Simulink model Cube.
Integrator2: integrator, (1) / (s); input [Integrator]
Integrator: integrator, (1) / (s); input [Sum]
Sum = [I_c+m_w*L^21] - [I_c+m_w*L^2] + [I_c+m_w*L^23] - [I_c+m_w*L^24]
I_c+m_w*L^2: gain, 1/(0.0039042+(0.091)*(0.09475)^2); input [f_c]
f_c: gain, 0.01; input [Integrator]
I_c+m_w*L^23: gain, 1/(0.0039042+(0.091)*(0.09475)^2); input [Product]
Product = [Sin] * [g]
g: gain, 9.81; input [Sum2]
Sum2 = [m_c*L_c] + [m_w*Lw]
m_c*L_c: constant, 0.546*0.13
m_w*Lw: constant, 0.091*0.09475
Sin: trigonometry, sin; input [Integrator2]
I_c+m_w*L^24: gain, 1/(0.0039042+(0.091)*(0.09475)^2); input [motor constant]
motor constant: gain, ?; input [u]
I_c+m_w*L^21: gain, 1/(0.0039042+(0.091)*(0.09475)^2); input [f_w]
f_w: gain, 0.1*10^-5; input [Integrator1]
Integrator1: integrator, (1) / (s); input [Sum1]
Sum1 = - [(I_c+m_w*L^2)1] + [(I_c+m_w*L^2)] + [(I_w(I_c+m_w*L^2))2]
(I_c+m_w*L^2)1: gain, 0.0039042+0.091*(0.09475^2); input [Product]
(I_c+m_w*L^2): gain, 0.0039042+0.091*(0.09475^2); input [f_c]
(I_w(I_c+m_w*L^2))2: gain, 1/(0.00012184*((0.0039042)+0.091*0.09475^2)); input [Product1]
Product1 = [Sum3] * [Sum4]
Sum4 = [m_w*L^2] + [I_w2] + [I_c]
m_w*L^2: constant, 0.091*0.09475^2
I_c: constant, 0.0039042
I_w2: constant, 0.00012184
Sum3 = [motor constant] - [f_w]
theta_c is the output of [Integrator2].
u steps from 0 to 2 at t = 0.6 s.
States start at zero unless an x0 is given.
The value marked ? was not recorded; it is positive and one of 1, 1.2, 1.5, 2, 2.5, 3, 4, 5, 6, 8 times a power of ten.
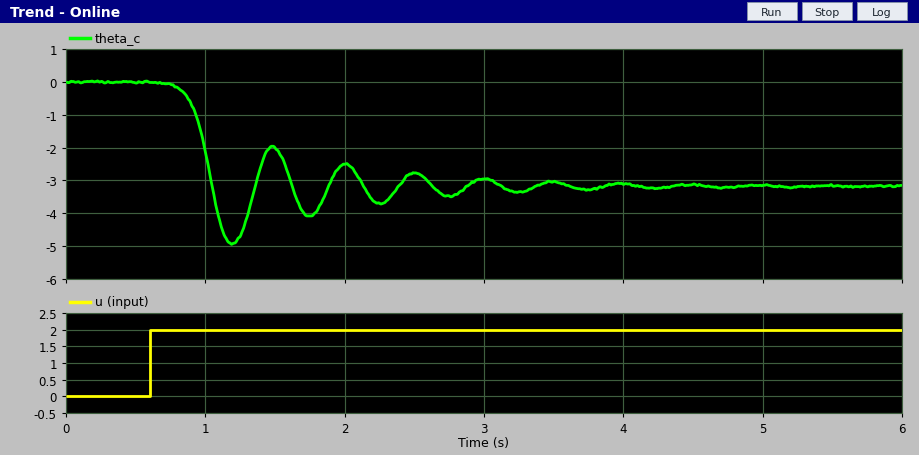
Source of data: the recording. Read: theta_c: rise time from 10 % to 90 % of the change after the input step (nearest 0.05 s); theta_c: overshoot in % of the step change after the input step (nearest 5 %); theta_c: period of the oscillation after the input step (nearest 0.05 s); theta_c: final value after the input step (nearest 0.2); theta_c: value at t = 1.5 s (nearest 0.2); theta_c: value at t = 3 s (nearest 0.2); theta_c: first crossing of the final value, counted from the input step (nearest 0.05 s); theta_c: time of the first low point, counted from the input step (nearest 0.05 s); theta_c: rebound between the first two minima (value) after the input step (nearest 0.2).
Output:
0.20 s
55 %
0.55 s
-3.2
-2.0
-3.0
0.45 s
0.60 s
-2.0
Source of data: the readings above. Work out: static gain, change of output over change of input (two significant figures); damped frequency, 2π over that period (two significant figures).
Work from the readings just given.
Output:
-1.6
11 rad/s
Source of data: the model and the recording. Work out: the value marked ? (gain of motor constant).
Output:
0.015
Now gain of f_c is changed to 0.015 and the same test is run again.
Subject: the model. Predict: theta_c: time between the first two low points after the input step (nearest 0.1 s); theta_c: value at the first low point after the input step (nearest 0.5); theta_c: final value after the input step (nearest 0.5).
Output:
0.5 s
-4.5
-3.0
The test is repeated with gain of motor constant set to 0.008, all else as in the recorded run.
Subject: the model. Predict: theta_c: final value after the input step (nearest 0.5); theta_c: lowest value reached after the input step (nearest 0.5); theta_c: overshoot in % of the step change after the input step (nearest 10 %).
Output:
-3.0
-5.0
50 %
